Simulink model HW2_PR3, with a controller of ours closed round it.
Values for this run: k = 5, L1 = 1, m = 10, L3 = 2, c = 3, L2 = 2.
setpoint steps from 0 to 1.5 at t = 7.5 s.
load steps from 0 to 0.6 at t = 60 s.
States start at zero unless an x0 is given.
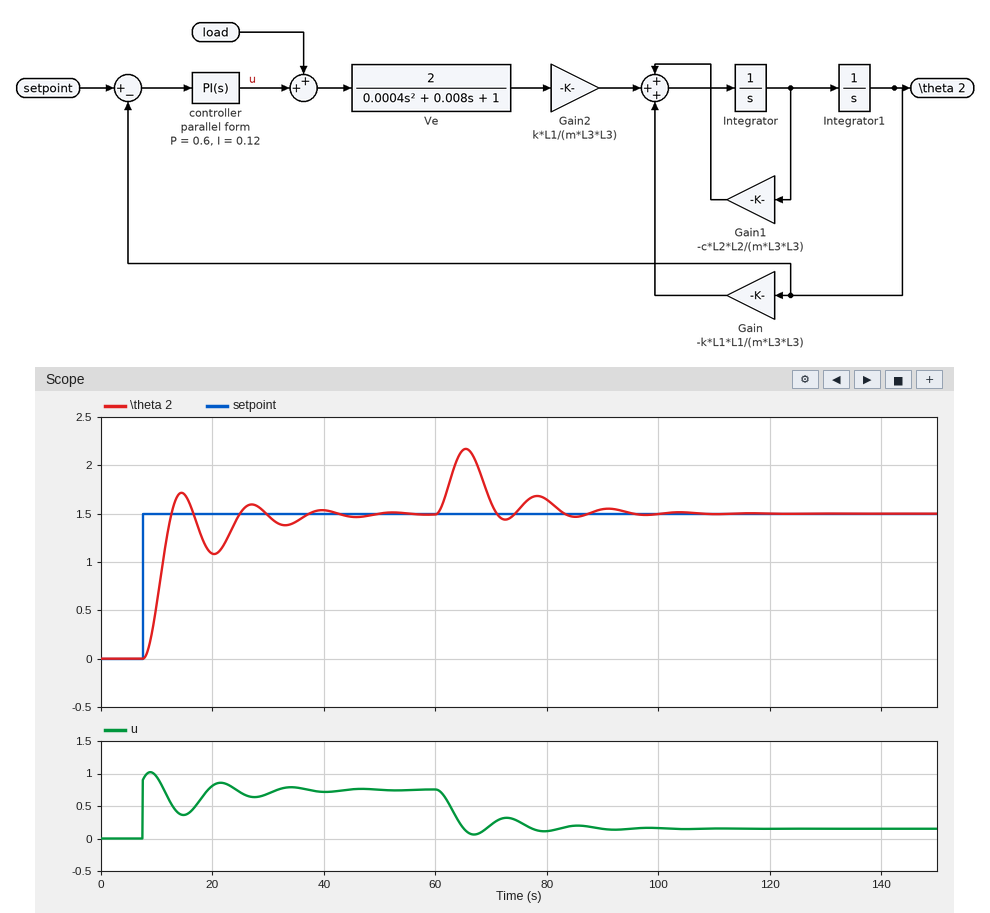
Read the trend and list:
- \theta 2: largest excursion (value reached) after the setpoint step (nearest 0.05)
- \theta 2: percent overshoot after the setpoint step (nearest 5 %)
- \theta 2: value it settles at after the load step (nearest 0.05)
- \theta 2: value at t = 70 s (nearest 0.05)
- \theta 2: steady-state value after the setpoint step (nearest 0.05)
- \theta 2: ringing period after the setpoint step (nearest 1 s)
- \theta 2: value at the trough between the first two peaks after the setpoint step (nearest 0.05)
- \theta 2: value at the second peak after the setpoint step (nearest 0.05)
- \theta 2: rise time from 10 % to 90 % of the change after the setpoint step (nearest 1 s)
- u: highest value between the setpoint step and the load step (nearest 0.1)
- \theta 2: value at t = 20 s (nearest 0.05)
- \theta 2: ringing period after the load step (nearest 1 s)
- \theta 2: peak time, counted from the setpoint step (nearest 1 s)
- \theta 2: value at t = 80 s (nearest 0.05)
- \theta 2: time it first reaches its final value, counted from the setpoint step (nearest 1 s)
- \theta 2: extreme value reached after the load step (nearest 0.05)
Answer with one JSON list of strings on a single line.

["1.70", "15 %", "1.50", "1.60", "1.50", "13 s", "1.10", "1.60", "3 s", "1.0", "1.10", "13 s", "7 s", "1.65", "5 s", "2.15"]
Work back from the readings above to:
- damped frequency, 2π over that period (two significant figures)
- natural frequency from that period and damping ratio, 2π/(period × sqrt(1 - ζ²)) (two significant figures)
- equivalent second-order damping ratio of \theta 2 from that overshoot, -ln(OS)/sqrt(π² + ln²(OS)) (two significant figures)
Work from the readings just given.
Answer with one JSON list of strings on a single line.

["0.48 rad/s", "0.57 rad/s", "0.52"]
